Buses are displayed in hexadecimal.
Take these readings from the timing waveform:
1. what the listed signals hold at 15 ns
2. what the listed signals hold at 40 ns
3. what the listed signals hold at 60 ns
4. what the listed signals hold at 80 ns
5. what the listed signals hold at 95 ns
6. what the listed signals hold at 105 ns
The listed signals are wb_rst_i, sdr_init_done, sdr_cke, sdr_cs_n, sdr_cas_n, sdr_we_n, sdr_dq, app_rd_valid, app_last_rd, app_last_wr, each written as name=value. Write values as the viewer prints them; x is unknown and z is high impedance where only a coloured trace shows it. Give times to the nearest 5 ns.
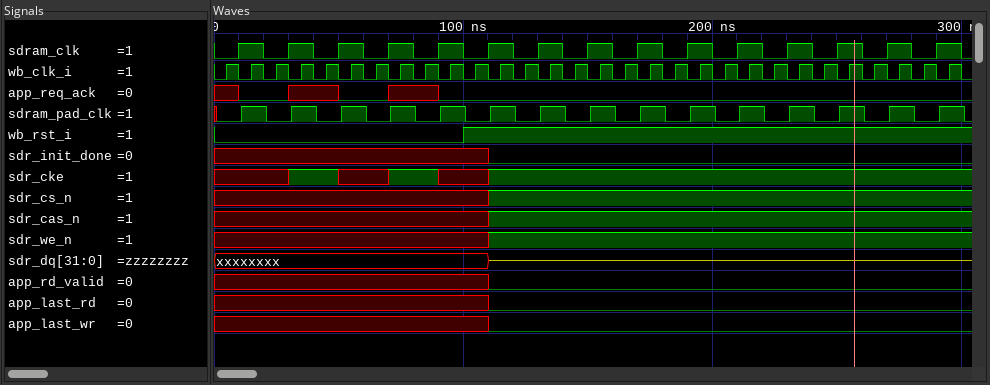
wb_rst_i=0, sdr_init_done=x, sdr_cke=x, sdr_cs_n=x, sdr_cas_n=x, sdr_we_n=x, sdr_dq=xxxxxxxx, app_rd_valid=x, app_last_rd=x, app_last_wr=x
wb_rst_i=0, sdr_init_done=x, sdr_cke=1, sdr_cs_n=x, sdr_cas_n=x, sdr_we_n=x, sdr_dq=xxxxxxxx, app_rd_valid=x, app_last_rd=x, app_last_wr=x
wb_rst_i=0, sdr_init_done=x, sdr_cke=x, sdr_cs_n=x, sdr_cas_n=x, sdr_we_n=x, sdr_dq=xxxxxxxx, app_rd_valid=x, app_last_rd=x, app_last_wr=x
wb_rst_i=0, sdr_init_done=x, sdr_cke=1, sdr_cs_n=x, sdr_cas_n=x, sdr_we_n=x, sdr_dq=xxxxxxxx, app_rd_valid=x, app_last_rd=x, app_last_wr=x
wb_rst_i=0, sdr_init_done=x, sdr_cke=x, sdr_cs_n=x, sdr_cas_n=x, sdr_we_n=x, sdr_dq=xxxxxxxx, app_rd_valid=x, app_last_rd=x, app_last_wr=x
wb_rst_i=1, sdr_init_done=x, sdr_cke=x, sdr_cs_n=x, sdr_cas_n=x, sdr_we_n=x, sdr_dq=xxxxxxxx, app_rd_valid=x, app_last_rd=x, app_last_wr=x
